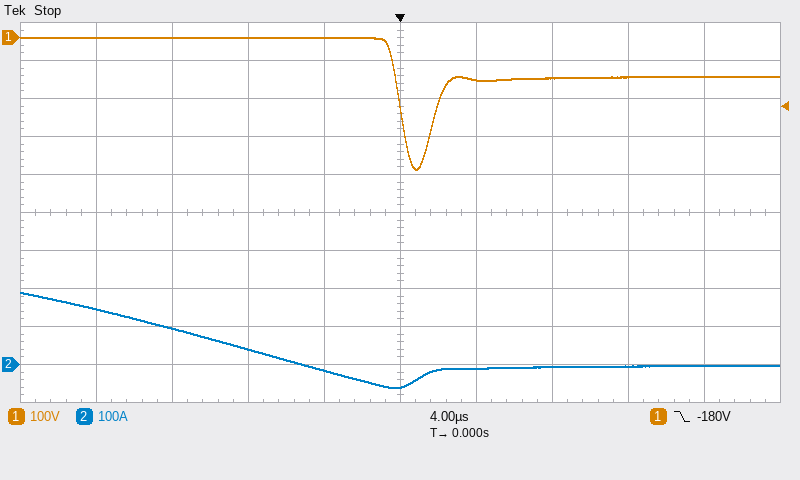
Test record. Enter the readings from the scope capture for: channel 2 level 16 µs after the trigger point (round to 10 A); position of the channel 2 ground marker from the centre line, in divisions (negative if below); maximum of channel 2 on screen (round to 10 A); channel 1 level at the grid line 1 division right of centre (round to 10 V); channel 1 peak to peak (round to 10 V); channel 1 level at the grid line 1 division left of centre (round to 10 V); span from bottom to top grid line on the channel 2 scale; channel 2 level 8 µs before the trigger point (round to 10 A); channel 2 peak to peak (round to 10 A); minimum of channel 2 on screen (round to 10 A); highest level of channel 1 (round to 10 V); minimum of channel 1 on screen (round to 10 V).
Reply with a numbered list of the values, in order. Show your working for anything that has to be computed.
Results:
1. 0 A
2. -4.0 div
3. 190 A
4. -110 V
5. 0 V − (-350 V) = 350 V
6. 0 V
7. 1 kA
8. 40 A
9. 190 A − (-60 A) = 250 A
10. -60 A
11. 0 V
12. -350 V
